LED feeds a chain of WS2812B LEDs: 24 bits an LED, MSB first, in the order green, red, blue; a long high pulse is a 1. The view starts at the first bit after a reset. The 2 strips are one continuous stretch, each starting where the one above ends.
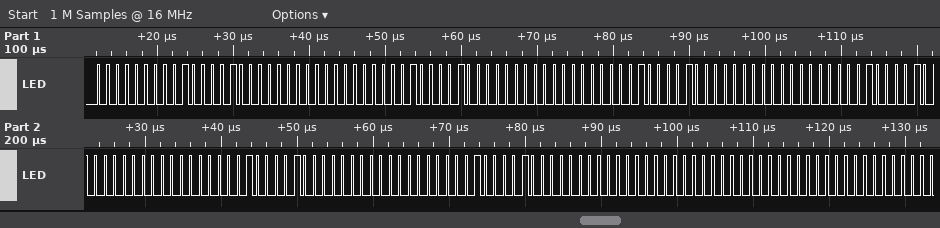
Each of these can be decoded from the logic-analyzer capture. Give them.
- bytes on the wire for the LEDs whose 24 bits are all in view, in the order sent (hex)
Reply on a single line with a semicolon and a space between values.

00 42 00 00 42 00 00 42 00 00 42 00 00 42 00 00 42 00 00 00 00
